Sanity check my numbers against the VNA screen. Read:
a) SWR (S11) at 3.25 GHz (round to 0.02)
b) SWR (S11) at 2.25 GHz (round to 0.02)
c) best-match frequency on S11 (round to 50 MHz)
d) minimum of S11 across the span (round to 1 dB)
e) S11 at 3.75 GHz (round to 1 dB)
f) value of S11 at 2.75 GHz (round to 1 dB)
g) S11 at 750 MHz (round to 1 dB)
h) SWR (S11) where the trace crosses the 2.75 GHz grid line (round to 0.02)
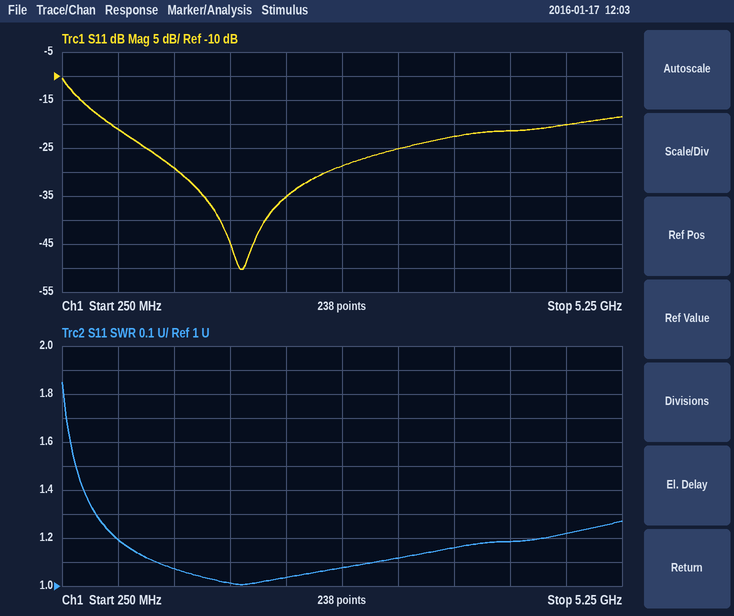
1.12
1.04
1.85 GHz
-50 dB
-23 dB
-29 dB
-21 dB
1.08
